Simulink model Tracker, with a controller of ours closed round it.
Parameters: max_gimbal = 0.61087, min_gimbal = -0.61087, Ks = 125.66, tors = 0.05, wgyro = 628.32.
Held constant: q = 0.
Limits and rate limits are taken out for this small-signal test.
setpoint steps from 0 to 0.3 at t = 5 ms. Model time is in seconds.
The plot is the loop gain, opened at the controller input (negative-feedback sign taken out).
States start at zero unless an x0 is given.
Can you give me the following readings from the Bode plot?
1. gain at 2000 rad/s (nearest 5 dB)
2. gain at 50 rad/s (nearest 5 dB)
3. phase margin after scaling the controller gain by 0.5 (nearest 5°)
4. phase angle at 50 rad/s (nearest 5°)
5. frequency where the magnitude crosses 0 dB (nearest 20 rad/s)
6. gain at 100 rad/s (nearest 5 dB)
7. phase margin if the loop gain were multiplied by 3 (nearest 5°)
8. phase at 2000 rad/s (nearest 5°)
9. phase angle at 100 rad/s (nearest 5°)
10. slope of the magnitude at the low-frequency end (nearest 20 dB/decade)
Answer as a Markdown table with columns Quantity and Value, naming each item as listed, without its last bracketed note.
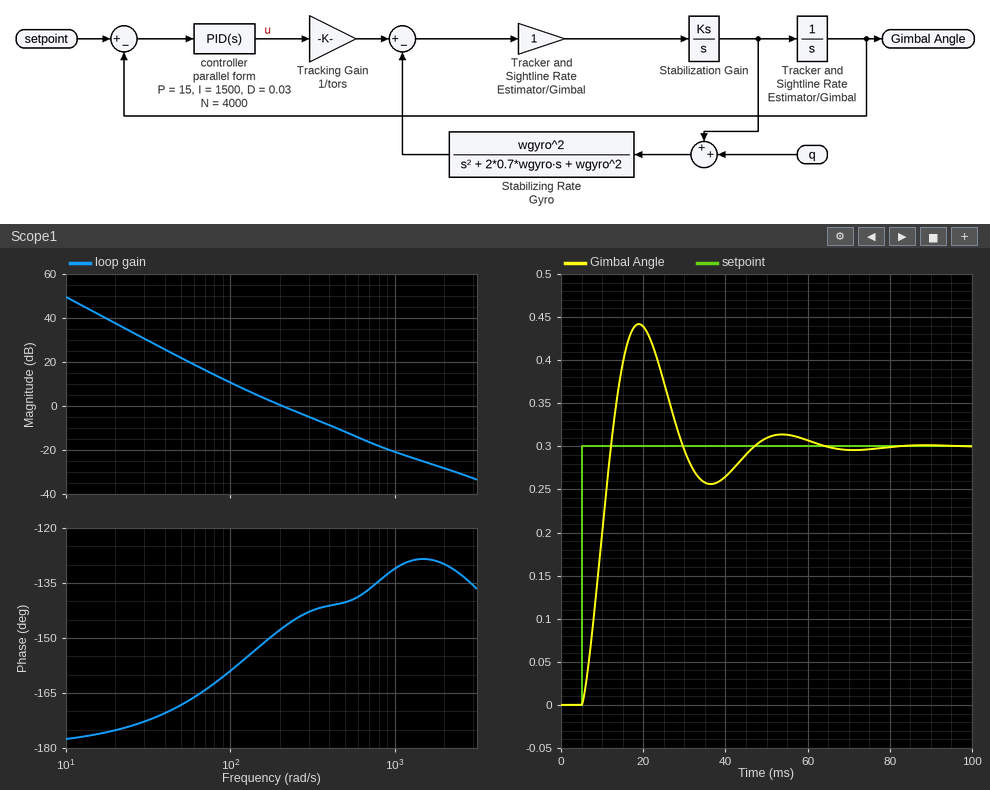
| Quantity | Value |
|---|---|
| gain at 2000 rad/s | -30 dB |
| gain at 50 rad/s | 20 dB |
| phase margin after scaling the controller gain by 0.5 | 25° |
| phase angle at 50 rad/s | -170° |
| frequency where the magnitude crosses 0 dB | 200 rad/s |
| gain at 100 rad/s | 10 dB |
| phase margin if the loop gain were multiplied by 3 | 40° |
| phase at 2000 rad/s | -130° |
| phase angle at 100 rad/s | -160° |
| slope of the magnitude at the low-frequency end | -40 dB/decade |
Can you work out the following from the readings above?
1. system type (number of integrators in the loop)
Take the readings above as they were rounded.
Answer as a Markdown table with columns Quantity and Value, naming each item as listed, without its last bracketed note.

| Quantity | Value |
|---|---|
| system type | 2 |
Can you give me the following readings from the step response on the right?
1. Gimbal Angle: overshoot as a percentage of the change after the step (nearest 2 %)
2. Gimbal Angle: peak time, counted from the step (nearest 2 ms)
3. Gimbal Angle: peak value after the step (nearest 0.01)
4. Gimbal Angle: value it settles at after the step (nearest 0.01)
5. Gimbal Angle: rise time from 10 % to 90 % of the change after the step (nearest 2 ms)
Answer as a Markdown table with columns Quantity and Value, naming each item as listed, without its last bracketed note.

| Quantity | Value |
|---|---|
| Gimbal Angle: overshoot as a percentage of the change after the step | 48 % |
| Gimbal Angle: peak time, counted from the step | 14 ms |
| Gimbal Angle: peak value after the step | 0.44 |
| Gimbal Angle: value it settles at after the step | 0.30 |
| Gimbal Angle: rise time from 10 % to 90 % of the change after the step | 6 ms |
